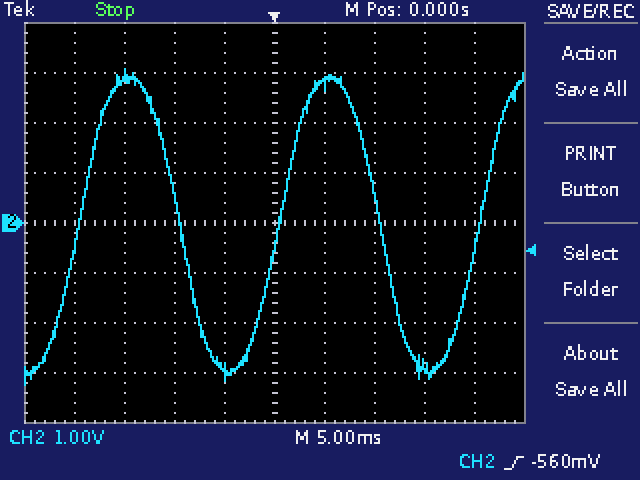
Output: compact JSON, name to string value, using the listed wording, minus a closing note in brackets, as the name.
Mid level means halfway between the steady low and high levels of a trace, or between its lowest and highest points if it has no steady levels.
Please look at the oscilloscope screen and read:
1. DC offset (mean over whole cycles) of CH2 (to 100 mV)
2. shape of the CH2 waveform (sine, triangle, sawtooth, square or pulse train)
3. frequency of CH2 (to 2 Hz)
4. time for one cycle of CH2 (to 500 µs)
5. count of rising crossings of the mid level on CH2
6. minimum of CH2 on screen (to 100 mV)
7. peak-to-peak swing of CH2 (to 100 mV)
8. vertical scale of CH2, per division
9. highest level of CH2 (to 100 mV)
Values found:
{"DC offset (mean over whole cycles) of CH2": "0.0 V", "shape of the CH2 waveform": "sine", "frequency of CH2": "50 Hz", "time for one cycle of CH2": "20.0 ms", "count of rising crossings of the mid level on CH2": "3", "minimum of CH2 on screen": "-3.2 V", "peak-to-peak swing of CH2": "6.3 V", "vertical scale of CH2, per division": "1 V", "highest level of CH2": "3.1 V"}
